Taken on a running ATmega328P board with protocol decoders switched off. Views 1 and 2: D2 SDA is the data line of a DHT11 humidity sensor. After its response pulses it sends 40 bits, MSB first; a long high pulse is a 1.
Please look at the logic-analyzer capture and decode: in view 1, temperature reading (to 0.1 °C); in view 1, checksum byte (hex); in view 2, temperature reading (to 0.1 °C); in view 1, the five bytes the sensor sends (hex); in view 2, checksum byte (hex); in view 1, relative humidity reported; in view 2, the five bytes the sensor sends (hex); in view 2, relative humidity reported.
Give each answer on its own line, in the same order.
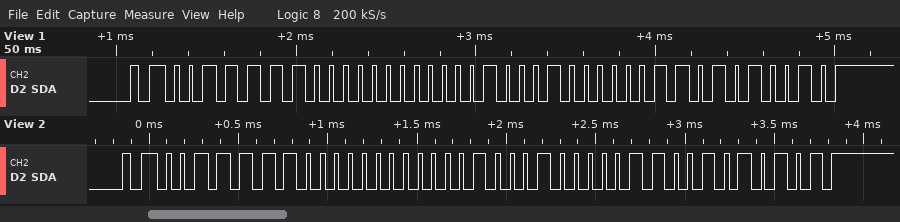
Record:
17.3 °C
0x52
17.6 °C
3E 00 11 03 52
0x55
62 %
3E 00 11 06 55
62 %
